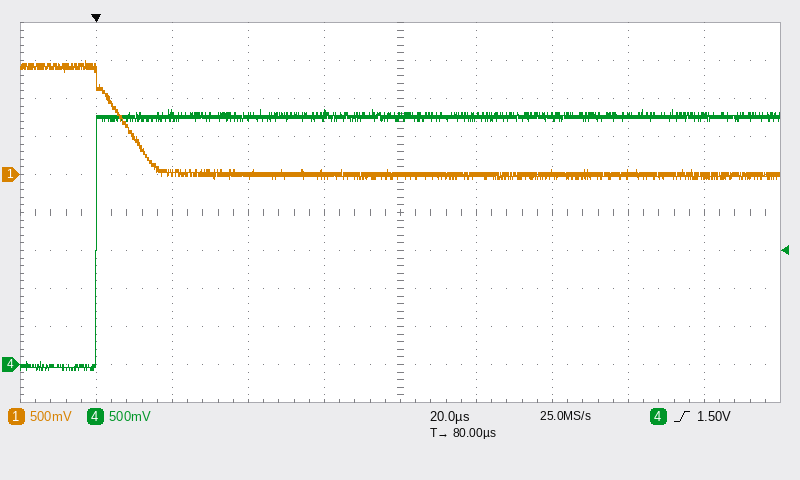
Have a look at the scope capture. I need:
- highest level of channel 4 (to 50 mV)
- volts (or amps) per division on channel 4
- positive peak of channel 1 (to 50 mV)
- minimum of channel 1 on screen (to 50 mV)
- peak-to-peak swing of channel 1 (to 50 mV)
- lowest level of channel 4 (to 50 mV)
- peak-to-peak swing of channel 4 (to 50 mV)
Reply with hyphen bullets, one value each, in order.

- 3.35 V
- 500 mV
- 1.50 V
- -50 mV
- 1.55 V
- -100 mV
- 3.45 V
